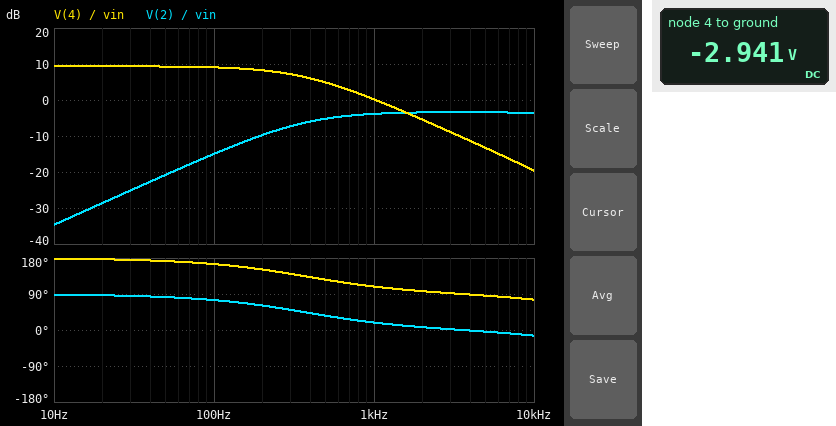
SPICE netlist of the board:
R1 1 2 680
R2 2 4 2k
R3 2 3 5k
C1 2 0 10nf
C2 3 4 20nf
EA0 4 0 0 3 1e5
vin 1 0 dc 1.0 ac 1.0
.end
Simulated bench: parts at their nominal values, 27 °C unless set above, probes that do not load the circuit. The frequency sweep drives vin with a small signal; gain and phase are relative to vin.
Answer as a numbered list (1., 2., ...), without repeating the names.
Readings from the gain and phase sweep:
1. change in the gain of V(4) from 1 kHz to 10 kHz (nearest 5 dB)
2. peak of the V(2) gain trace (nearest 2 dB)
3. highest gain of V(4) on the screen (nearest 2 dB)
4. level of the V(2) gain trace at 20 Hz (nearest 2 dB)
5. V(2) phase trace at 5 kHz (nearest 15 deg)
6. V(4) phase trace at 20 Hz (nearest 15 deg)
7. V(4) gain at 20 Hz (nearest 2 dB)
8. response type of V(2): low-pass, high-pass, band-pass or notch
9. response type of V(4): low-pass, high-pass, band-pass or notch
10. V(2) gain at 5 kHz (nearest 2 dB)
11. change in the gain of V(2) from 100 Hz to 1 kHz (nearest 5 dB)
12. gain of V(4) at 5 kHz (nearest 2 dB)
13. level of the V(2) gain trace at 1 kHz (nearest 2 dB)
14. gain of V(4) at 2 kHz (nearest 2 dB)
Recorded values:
1. -20 dB
2. -4 dB
3. 10 dB
4. -28 dB
5. 0 deg
6. 180 deg
7. 10 dB
8. high-pass
9. low-pass
10. -4 dB
11. 10 dB
12. -14 dB
13. -4 dB
14. -6 dB
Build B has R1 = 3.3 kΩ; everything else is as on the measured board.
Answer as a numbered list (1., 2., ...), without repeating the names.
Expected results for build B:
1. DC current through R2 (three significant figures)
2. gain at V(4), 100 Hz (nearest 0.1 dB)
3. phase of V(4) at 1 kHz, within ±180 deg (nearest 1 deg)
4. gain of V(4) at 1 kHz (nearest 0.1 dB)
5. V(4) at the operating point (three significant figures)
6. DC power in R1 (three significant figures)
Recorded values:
1. 303 µA
2. -4.4 dB
3. 126 deg
4. -8.2 dB
5. -606 mV
6. 303 µW
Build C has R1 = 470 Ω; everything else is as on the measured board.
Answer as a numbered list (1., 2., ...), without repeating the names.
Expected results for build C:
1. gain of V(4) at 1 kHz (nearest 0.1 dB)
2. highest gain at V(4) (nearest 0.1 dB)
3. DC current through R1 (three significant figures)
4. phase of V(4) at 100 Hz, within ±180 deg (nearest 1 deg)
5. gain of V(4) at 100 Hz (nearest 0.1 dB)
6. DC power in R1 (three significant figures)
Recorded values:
1. 1.3 dB
2. 12.6 dB
3. 2.13 mA
4. 160 deg
5. 12.1 dB
6. 2.13 mW
